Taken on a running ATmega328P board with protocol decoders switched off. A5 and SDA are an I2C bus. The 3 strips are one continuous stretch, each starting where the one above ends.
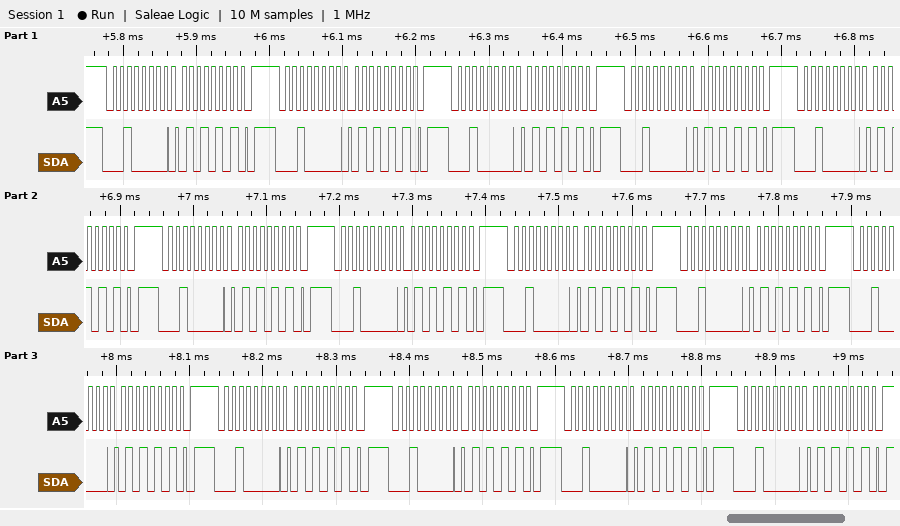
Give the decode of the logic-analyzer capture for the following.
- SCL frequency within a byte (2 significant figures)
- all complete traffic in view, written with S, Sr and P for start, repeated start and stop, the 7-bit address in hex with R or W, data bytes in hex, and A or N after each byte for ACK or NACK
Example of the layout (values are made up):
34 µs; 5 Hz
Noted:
100 kHz; S 10W A 55 A P S 10W A 55 A P S 10W A 55 A P S 10W A 55 A P S 10W A 55 A P S 10W A 55 A P S 10W A 55 A P S 10W A 55 A P S 10W A 55 A P S 10W A 55 A P S 10W A 55 A P S 10W A 55 A P S 10W A 55 A P S 10W A 55 A P
